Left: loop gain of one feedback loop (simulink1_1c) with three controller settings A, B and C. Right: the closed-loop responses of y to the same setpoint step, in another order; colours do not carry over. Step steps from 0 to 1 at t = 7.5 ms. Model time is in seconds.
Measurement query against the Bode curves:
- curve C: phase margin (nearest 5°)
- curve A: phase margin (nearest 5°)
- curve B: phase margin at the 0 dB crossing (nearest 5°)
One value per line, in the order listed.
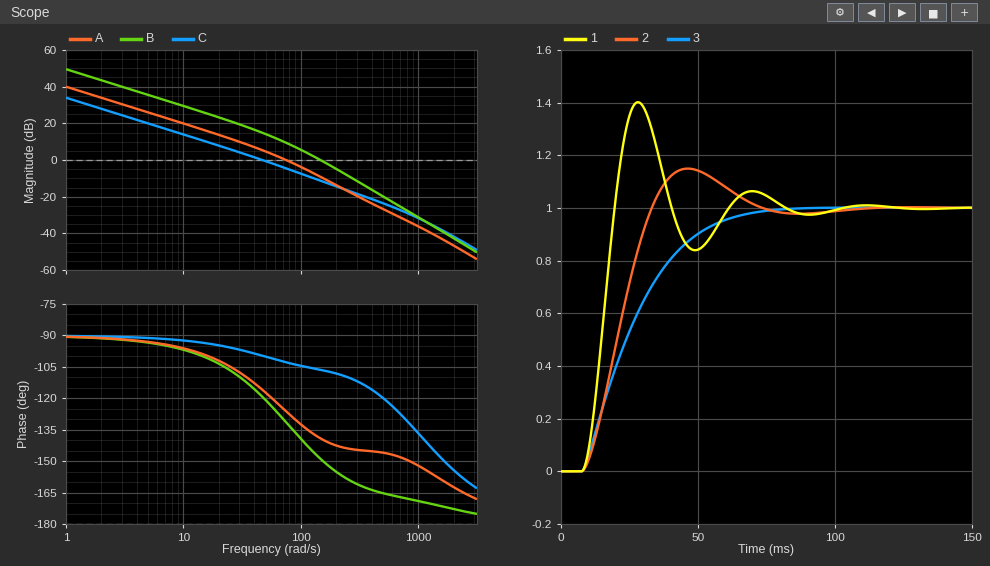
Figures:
80°
55°
30°
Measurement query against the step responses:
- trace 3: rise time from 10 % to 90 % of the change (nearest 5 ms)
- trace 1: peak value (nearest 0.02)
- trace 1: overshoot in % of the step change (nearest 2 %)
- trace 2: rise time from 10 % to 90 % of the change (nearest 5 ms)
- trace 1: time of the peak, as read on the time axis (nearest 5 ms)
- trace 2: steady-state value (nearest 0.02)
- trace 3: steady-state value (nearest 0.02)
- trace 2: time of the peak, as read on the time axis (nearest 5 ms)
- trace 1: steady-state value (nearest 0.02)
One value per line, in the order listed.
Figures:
40 ms
1.40
40 %
20 ms
30 ms
1.00
1.00
45 ms
1.00
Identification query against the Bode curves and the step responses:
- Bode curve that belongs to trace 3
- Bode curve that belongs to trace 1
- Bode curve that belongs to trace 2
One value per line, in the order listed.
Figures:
C
B
A
